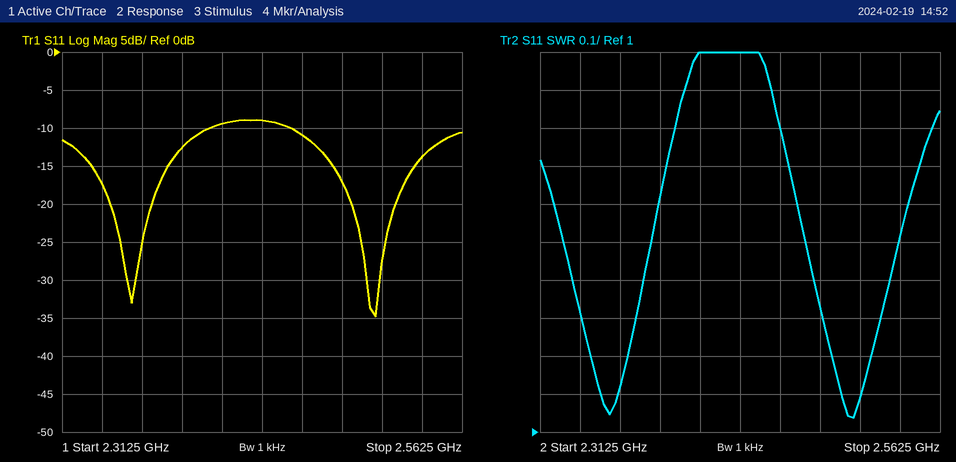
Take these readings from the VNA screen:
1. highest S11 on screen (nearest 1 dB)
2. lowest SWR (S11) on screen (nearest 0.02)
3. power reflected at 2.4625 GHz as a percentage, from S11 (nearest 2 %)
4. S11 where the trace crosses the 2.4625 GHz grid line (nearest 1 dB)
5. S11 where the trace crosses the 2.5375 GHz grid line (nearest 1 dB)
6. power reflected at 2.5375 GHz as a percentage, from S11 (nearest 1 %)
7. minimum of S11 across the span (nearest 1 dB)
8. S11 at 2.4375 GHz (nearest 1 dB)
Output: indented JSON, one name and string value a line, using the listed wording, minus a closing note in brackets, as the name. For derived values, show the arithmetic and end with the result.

{
  "highest S11 on screen": "-9 dB",
  "lowest SWR (S11) on screen": "1.04",
  "power reflected at 2.4625 GHz as a percentage, from S11": "10^(-11/10) ≈ 8 %",
  "S11 where the trace crosses the 2.4625 GHz grid line": "-11 dB",
  "S11 where the trace crosses the 2.5375 GHz grid line": "-14 dB",
  "power reflected at 2.5375 GHz as a percentage, from S11": "10^(-14/10) ≈ 4 %",
  "minimum of S11 across the span": "-35 dB",
  "S11 at 2.4375 GHz": "-9 dB"
}
